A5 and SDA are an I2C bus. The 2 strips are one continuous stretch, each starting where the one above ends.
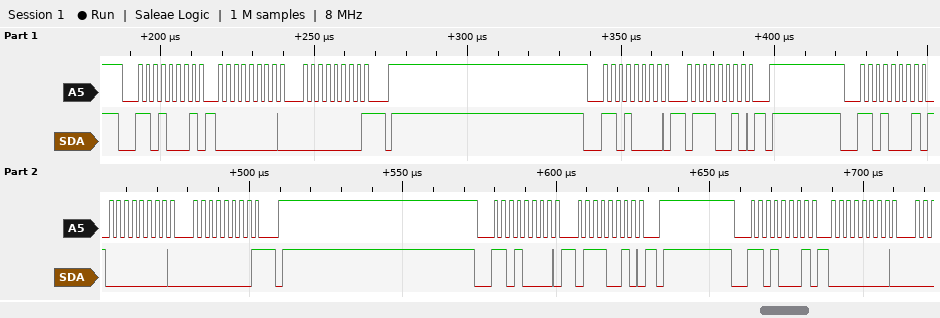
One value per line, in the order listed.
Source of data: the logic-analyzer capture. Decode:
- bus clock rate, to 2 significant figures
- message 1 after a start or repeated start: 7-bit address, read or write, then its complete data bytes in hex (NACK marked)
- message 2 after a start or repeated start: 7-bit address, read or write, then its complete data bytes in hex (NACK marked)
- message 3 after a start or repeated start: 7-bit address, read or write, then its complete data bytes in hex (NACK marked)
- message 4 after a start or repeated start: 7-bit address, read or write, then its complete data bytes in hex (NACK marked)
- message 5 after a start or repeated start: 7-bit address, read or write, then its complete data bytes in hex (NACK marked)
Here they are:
400 kHz
0x68 read: 00 00 NACK
0x68 write: 72
0x68 read: 00 00 NACK
0x68 write: 72
0x68 read: 00
